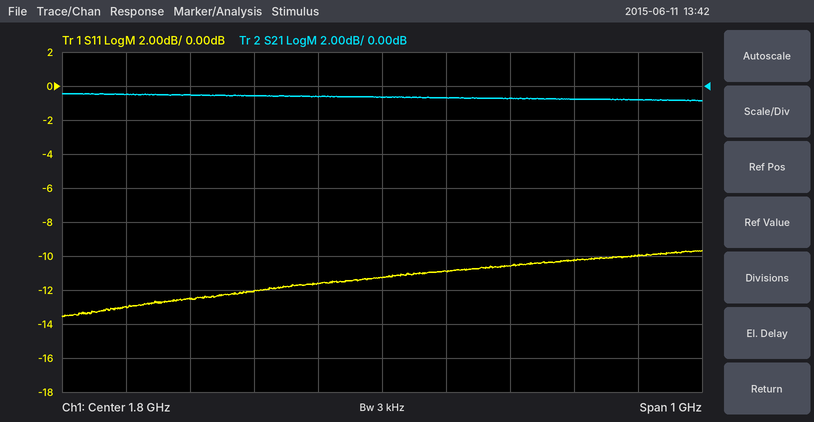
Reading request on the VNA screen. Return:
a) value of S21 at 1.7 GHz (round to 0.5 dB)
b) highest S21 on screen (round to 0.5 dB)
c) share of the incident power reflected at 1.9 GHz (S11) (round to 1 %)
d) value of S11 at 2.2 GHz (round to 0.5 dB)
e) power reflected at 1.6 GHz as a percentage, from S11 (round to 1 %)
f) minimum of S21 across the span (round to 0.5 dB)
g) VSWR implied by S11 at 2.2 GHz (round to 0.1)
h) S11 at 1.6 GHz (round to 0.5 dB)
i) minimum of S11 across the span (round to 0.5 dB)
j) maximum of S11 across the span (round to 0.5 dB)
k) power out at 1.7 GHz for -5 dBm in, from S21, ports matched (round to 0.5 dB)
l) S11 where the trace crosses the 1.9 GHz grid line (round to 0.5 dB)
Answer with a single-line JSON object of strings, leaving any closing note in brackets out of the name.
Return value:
{"value of S21 at 1.7 GHz": "-0.5 dB", "highest S21 on screen": "-0.5 dB", "share of the incident power reflected at 1.9 GHz (S11)": "8 %", "value of S11 at 2.2 GHz": "-10.0 dB", "power reflected at 1.6 GHz as a percentage, from S11": "6 %", "minimum of S21 across the span": "-1.0 dB", "VSWR implied by S11 at 2.2 GHz": "1.9", "S11 at 1.6 GHz": "-12.0 dB", "minimum of S11 across the span": "-13.5 dB", "maximum of S11 across the span": "-9.5 dB", "power out at 1.7 GHz for -5 dBm in, from S21, ports matched": "-5.5 dBm", "S11 where the trace crosses the 1.9 GHz grid line": "-11.0 dB"}
